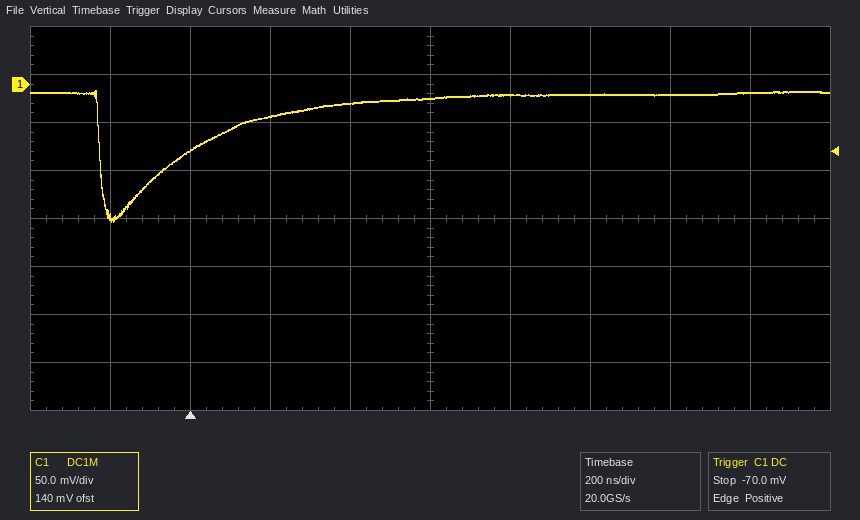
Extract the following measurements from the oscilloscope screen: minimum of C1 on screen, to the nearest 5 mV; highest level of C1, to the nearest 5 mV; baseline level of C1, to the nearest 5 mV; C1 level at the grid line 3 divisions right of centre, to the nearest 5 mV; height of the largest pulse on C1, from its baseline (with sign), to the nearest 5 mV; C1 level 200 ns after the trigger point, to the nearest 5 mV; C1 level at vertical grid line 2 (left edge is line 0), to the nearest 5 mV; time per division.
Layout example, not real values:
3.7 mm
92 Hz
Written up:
-145 mV
-5 mV
-10 mV
-10 mV
-135 mV
-35 mV
-70 mV
200 ns
